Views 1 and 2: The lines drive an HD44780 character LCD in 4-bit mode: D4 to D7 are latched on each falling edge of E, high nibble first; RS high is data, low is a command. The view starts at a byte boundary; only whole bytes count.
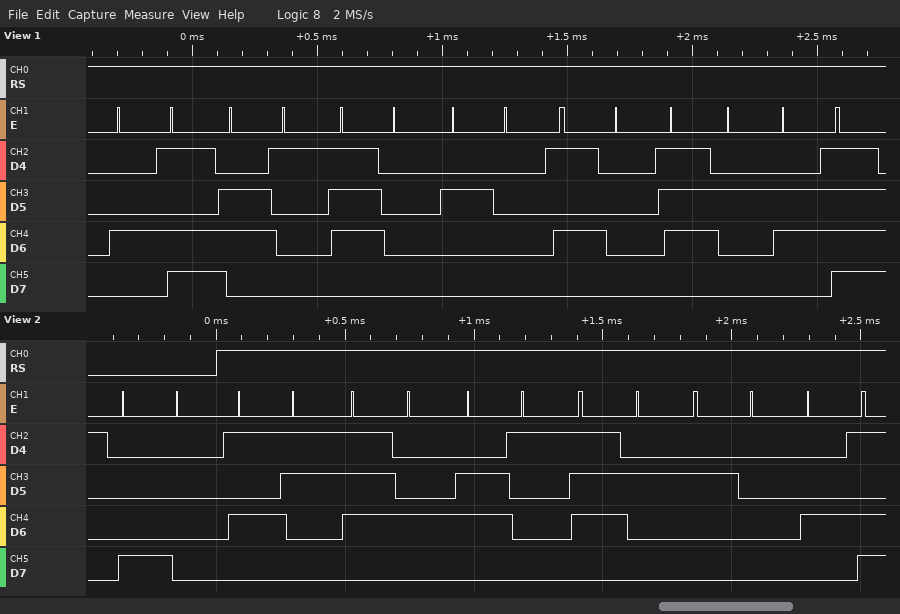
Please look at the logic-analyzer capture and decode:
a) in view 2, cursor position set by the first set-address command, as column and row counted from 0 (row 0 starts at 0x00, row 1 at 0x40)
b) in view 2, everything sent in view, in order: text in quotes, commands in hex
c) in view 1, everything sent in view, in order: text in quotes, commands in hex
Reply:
column 0, row 0
0x80 "Star M"
"Map Pro"
